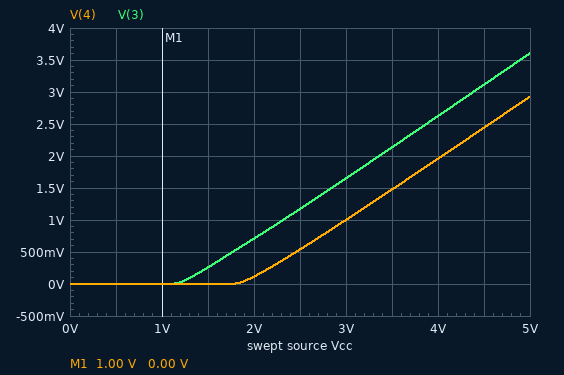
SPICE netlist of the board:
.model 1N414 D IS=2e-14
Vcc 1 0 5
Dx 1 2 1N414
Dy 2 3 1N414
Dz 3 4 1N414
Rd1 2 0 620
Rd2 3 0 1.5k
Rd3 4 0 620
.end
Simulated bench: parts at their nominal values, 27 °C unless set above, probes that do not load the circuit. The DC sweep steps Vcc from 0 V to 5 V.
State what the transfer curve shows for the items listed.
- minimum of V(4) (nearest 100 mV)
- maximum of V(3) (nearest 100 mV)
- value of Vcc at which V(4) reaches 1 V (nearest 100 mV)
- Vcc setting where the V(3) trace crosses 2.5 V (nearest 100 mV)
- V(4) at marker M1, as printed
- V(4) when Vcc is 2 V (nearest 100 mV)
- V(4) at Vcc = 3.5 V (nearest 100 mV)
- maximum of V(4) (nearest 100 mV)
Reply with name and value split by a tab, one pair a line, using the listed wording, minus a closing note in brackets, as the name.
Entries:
minimum of V(4)	0 V
maximum of V(3)	3.6 V
value of Vcc at which V(4) reaches 1 V	3.0 V
Vcc setting where the V(3) trace crosses 2.5 V	3.9 V
V(4) at marker M1, as printed	0.00 V
V(4) when Vcc is 2 V	100 mV
V(4) at Vcc = 3.5 V	1.5 V
maximum of V(4)	2.9 V
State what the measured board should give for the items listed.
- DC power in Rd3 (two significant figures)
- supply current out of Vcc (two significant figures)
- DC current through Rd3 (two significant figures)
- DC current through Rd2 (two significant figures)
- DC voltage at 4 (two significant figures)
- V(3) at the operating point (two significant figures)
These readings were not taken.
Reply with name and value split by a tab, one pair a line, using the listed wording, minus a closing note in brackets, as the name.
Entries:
DC power in Rd3	14 mW
supply current out of Vcc	14 mA
DC current through Rd3	4.7 mA
DC current through Rd2	2.4 mA
DC voltage at 4	2.9 V
V(3) at the operating point	3.6 V
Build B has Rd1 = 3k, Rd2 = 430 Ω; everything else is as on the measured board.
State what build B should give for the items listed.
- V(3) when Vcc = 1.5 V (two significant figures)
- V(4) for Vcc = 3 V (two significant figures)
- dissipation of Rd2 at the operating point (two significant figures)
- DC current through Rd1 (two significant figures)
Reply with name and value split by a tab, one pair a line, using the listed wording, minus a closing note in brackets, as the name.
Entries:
V(3) when Vcc = 1.5 V	240 mV
V(4) for Vcc = 3 V	990 mV
dissipation of Rd2 at the operating point	30 mW
DC current through Rd1	1.4 mA
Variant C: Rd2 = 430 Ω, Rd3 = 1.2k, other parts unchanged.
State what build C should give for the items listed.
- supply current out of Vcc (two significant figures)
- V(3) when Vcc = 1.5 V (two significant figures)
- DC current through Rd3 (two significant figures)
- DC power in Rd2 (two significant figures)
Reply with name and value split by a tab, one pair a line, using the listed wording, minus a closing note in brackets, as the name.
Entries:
supply current out of Vcc	18 mA
V(3) when Vcc = 1.5 V	230 mV
DC current through Rd3	2.4 mA
DC power in Rd2	30 mW
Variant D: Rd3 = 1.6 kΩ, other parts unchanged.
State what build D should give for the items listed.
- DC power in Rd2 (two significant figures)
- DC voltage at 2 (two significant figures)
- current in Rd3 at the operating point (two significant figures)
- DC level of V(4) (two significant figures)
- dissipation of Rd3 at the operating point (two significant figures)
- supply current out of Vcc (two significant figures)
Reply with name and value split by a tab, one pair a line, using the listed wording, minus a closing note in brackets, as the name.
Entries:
DC power in Rd2	8.8 mW
DC voltage at 2	4.3 V
current in Rd3 at the operating point	1.9 mA
DC level of V(4)	3.0 V
dissipation of Rd3 at the operating point	5.5 mW
supply current out of Vcc	11 mA
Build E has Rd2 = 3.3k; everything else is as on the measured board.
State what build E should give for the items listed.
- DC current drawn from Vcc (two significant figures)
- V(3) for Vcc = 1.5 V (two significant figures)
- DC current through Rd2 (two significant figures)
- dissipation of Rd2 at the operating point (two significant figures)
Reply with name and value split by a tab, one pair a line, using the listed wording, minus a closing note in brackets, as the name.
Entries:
DC current drawn from Vcc	13 mA
V(3) for Vcc = 1.5 V	280 mV
DC current through Rd2	1.1 mA
dissipation of Rd2 at the operating point	4.0 mW
